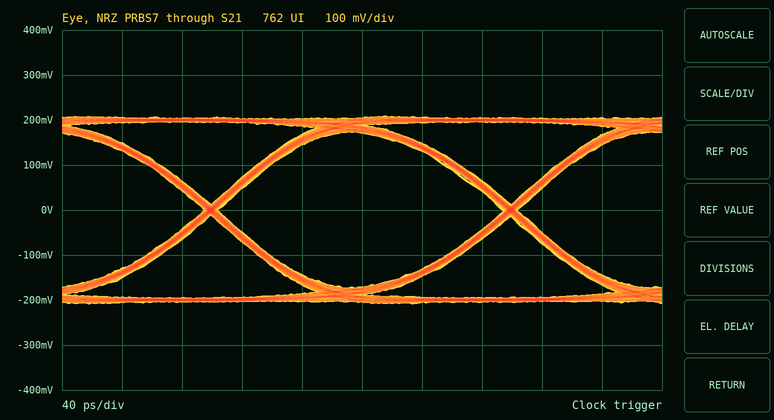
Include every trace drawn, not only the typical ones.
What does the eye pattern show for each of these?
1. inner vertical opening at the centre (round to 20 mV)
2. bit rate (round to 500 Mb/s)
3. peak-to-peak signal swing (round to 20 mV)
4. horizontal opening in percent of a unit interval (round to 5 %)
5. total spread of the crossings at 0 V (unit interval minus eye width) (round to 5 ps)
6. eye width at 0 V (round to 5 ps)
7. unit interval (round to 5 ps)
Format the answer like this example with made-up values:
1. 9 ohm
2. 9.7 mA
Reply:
1. 340 mV
2. 5.0 Gb/s
3. 420 mV
4. 95 %
5. 10 ps
6. 190 ps
7. 200 ps
